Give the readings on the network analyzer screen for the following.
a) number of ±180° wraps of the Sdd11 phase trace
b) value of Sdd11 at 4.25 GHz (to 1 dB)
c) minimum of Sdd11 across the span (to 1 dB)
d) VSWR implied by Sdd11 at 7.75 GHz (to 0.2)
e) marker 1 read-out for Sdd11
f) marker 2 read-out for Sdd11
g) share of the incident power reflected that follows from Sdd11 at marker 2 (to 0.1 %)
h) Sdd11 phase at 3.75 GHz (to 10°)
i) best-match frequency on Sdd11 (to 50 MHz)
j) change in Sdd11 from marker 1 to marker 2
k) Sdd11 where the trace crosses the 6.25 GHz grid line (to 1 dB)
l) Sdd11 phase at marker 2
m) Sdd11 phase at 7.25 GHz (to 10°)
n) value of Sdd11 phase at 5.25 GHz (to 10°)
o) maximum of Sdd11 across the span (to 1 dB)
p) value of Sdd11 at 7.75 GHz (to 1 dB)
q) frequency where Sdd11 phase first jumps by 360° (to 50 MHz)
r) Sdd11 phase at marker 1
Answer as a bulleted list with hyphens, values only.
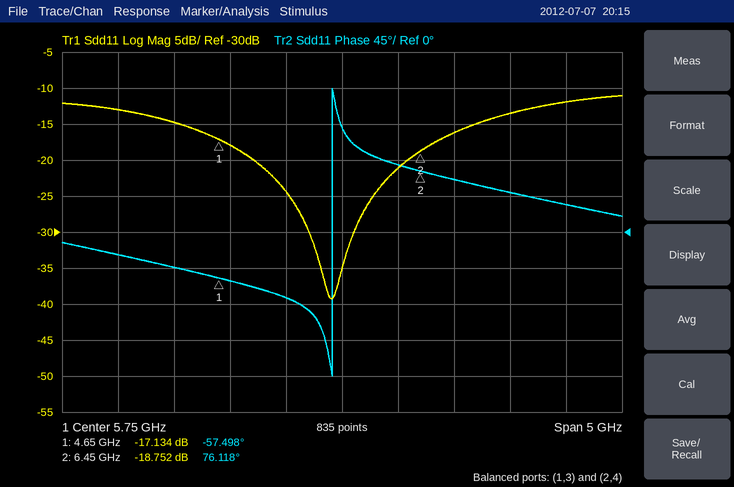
- 1
- -15 dB
- -39 dB
- 1.6
- -17.134 dB
- -18.752 dB
- 1.3 %
- -30°
- 5.65 GHz
- -1.618 dB
- -21 dB
- 76.118°
- 50°
- -80°
- -11 dB
- -12 dB
- 5.65 GHz
- -57.498°
